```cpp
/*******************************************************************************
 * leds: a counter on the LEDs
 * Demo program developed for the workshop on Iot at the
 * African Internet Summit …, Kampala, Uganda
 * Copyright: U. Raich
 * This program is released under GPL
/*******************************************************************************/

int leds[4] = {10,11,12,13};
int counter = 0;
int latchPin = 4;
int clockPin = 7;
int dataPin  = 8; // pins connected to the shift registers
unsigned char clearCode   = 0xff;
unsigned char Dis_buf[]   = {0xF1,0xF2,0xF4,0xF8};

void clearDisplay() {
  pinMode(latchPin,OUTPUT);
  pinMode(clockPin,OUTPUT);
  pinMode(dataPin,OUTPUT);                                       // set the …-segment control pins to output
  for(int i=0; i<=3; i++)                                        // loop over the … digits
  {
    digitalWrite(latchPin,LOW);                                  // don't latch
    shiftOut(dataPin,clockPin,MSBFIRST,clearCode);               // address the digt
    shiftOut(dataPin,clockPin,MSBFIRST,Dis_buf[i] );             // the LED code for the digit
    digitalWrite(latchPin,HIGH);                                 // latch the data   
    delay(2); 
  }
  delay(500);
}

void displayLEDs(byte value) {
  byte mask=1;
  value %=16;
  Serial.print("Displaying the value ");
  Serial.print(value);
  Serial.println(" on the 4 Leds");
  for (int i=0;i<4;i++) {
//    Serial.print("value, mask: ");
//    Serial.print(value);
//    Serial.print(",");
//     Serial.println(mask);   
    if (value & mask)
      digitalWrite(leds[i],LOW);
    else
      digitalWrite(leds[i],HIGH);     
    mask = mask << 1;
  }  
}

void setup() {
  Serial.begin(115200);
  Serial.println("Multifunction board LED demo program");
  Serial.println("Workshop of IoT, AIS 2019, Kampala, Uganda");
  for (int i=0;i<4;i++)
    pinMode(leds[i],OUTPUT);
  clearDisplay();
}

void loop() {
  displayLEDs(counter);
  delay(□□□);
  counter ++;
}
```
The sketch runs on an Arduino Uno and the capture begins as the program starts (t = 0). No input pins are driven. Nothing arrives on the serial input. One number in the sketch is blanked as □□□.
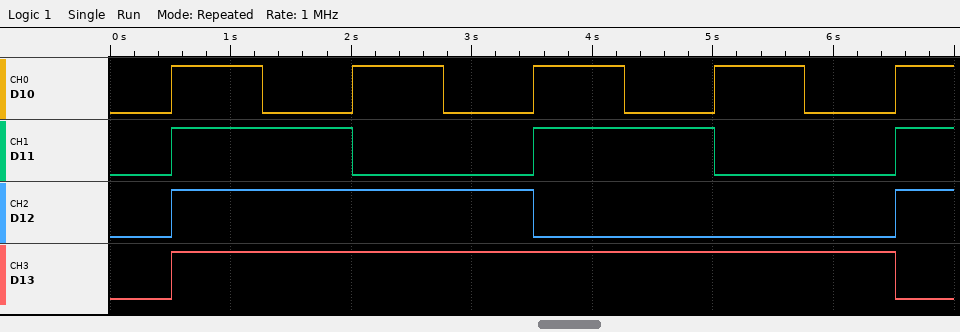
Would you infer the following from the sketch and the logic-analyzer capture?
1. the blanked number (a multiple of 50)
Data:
750
